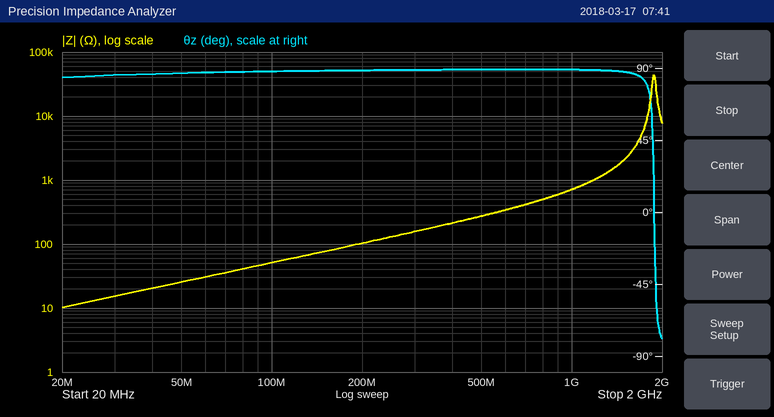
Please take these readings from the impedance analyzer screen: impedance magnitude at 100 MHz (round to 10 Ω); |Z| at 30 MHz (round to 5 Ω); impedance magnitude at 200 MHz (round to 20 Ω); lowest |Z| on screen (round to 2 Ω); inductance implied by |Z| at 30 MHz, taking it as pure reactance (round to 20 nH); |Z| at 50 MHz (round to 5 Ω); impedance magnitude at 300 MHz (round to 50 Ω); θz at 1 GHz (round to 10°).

50 Ω
15 Ω
100 Ω
10 Ω
80 nH
25 Ω
150 Ω
90°
